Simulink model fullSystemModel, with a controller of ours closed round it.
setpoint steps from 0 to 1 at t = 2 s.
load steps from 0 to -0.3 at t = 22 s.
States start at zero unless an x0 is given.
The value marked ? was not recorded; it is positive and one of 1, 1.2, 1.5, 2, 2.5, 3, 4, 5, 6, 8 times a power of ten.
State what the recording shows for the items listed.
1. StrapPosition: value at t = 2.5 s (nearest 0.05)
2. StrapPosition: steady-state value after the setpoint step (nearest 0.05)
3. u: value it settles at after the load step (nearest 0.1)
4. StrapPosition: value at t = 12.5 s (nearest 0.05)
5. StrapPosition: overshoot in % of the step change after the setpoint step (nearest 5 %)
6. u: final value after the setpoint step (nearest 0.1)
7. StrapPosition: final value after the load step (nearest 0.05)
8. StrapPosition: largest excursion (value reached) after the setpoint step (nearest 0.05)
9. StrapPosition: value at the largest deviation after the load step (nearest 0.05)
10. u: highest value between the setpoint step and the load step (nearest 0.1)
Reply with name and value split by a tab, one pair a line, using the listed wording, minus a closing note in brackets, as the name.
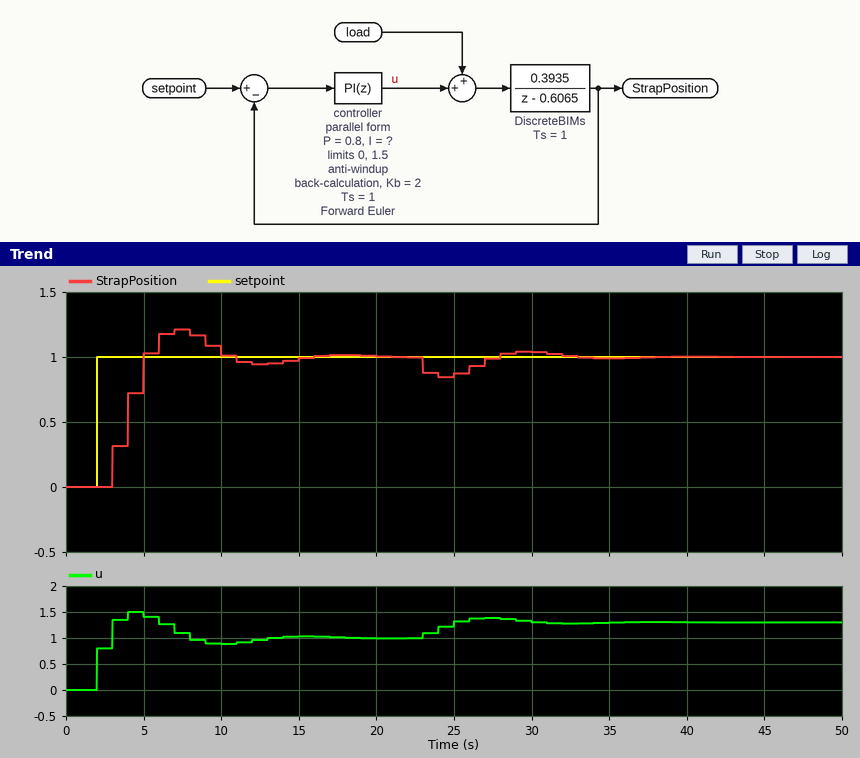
StrapPosition: value at t = 2.5 s	0.00
StrapPosition: steady-state value after the setpoint step	1.00
u: value it settles at after the load step	1.3
StrapPosition: value at t = 12.5 s	0.95
StrapPosition: overshoot in % of the step change after the setpoint step	20 %
u: final value after the setpoint step	1.0
StrapPosition: final value after the load step	1.00
StrapPosition: largest excursion (value reached) after the setpoint step	1.20
StrapPosition: value at the largest deviation after the load step	0.85
u: highest value between the setpoint step and the load step	1.5
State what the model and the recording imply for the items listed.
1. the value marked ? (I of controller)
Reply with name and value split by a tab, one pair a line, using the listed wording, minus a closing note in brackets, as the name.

the value marked ?	0.8
